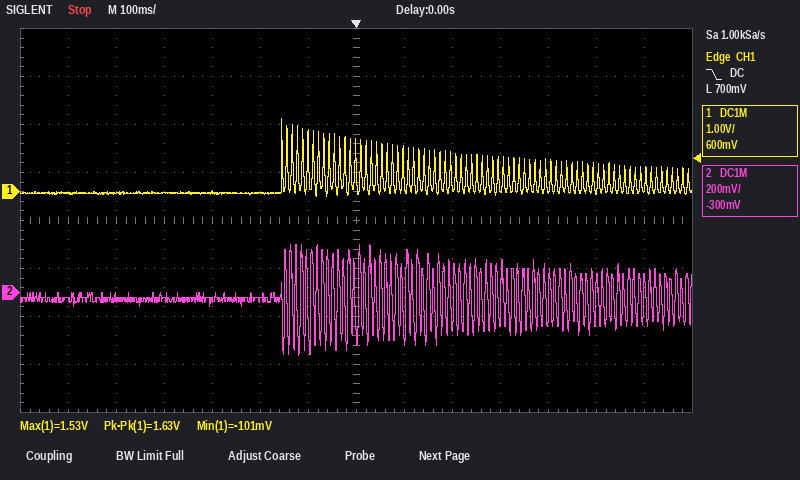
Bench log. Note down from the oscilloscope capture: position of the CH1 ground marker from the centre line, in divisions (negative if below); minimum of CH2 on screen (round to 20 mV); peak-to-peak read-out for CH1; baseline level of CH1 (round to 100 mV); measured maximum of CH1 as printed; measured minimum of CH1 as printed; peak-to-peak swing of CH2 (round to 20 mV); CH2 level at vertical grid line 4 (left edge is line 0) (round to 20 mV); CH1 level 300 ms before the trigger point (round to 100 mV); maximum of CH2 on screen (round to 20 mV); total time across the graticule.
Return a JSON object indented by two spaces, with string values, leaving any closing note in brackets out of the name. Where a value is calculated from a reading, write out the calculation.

{
  "position of the CH1 ground marker from the centre line, in divisions": "+0.6 div",
  "minimum of CH2 on screen": "-260 mV",
  "peak-to-peak read-out for CH1": "1.63 V",
  "baseline level of CH1": "0.0 V",
  "measured maximum of CH1 as printed": "1.53 V",
  "measured minimum of CH1 as printed": "-101 mV",
  "peak-to-peak swing of CH2": "200 mV − (-260 mV) = 460 mV",
  "CH2 level at vertical grid line 4 (left edge is line 0)": "-40 mV",
  "CH1 level 300 ms before the trigger point": "0.0 V",
  "maximum of CH2 on screen": "200 mV",
  "total time across the graticule": "1.4 s"
}
